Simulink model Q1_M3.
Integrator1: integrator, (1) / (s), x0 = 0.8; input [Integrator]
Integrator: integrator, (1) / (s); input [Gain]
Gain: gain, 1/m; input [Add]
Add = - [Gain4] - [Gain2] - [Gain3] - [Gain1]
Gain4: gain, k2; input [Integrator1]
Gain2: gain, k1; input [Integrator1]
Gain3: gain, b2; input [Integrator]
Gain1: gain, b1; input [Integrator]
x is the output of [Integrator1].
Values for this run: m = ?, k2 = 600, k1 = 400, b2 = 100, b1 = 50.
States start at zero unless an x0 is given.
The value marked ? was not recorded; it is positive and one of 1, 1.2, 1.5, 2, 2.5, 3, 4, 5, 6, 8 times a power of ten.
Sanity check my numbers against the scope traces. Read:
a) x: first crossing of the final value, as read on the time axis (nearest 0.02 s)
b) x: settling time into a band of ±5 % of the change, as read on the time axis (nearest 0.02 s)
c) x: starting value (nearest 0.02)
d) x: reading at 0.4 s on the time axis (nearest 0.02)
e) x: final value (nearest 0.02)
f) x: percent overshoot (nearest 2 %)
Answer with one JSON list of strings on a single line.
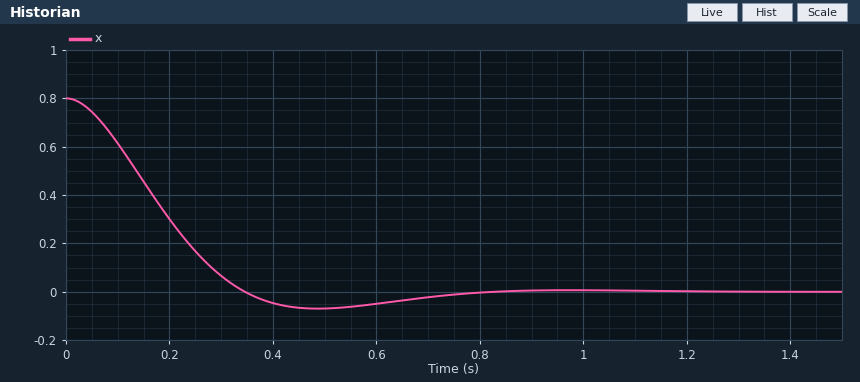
["0.34 s", "0.64 s", "0.80", "-0.04", "0.00", "8 %"]
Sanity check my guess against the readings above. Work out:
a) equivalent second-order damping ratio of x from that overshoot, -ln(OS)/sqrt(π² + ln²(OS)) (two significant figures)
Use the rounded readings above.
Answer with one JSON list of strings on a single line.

["0.63"]
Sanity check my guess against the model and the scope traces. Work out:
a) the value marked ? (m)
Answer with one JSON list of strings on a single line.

["15"]
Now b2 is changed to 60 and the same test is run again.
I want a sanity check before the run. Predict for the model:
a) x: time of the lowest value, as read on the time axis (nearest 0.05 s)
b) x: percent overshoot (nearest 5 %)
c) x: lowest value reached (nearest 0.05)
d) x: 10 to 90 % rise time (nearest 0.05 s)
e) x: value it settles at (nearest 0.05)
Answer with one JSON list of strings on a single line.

["0.45 s", "20 %", "-0.15", "0.20 s", "0.00"]
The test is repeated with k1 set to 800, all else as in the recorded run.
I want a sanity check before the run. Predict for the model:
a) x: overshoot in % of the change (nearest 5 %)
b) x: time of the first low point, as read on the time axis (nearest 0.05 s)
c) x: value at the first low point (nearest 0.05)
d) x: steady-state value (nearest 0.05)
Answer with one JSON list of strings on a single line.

["15 %", "0.40 s", "-0.10", "0.00"]
